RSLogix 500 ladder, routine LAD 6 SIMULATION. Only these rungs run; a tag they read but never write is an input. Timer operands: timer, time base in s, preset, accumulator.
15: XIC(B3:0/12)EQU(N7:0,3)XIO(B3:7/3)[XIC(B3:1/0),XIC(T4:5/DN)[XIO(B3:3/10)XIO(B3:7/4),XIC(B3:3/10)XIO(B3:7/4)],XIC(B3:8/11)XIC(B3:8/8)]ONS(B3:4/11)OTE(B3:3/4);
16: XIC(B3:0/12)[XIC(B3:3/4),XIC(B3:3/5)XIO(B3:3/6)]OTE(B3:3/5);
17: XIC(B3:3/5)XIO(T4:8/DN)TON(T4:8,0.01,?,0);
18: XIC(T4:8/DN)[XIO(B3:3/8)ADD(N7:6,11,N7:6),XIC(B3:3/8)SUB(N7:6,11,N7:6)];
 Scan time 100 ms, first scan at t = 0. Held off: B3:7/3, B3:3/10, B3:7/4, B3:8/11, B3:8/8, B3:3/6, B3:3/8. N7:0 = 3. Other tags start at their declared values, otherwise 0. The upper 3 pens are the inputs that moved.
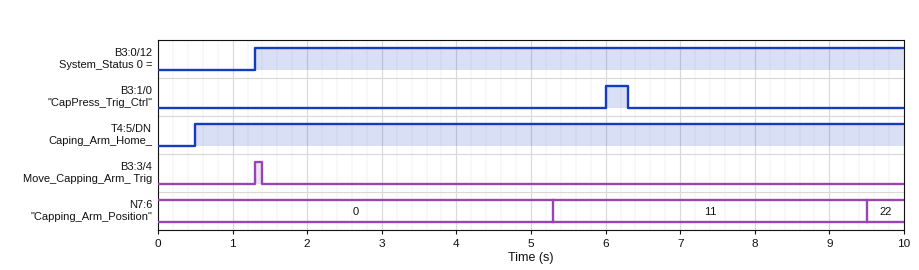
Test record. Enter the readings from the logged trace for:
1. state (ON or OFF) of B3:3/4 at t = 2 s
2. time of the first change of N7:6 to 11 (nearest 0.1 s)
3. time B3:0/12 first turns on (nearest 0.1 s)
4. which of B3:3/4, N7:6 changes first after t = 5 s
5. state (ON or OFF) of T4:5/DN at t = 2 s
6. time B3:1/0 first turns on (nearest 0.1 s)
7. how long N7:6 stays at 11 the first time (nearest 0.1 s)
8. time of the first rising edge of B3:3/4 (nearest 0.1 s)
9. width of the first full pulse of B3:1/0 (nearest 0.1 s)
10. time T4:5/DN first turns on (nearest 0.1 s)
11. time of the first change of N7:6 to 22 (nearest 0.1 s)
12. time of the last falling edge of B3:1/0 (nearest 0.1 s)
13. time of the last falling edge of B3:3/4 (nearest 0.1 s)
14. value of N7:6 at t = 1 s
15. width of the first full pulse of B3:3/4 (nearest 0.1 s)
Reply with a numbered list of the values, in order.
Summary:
1. OFF
2. 5.3 s
3. 1.3 s
4. N7:6
5. ON
6. 6.0 s
7. 4.2 s
8. 1.3 s
9. 0.3 s
10. 0.5 s
11. 9.5 s
12. 6.3 s
13. 1.4 s
14. 0
15. 0.1 s
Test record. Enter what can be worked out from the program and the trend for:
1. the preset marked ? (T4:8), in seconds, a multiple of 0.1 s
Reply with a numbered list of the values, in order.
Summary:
1. 4.0 s
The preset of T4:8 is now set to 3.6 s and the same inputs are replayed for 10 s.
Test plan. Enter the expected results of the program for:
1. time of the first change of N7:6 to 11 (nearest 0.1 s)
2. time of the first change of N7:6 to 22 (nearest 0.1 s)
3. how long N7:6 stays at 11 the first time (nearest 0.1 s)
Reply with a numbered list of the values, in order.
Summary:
1. 4.9 s
2. 8.7 s
3. 3.8 s
